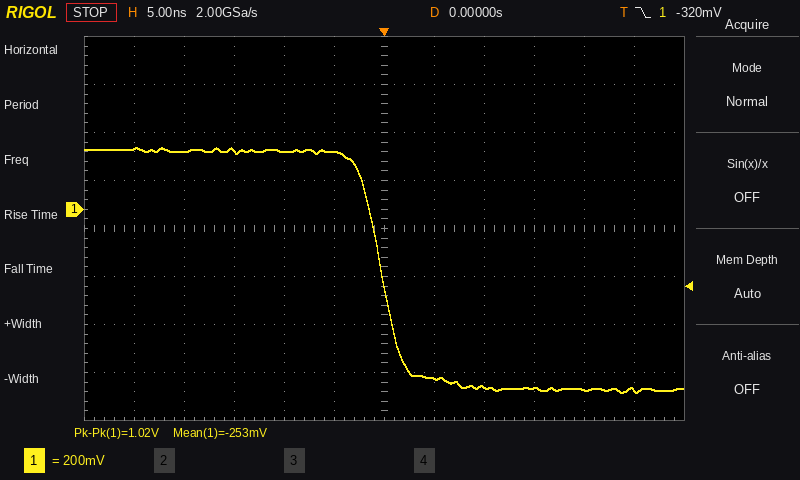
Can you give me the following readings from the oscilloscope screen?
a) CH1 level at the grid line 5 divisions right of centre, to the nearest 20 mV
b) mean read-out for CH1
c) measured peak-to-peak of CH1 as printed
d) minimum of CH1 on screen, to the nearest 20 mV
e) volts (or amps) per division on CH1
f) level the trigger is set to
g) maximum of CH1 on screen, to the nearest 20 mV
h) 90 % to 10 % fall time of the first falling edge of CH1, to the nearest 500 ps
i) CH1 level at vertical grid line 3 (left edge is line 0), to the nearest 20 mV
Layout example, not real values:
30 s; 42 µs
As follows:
-760 mV; -253 mV; 1.02 V; -760 mV; 200 mV; -320 mV; 260 mV; 4.5 ns; 240 mV
